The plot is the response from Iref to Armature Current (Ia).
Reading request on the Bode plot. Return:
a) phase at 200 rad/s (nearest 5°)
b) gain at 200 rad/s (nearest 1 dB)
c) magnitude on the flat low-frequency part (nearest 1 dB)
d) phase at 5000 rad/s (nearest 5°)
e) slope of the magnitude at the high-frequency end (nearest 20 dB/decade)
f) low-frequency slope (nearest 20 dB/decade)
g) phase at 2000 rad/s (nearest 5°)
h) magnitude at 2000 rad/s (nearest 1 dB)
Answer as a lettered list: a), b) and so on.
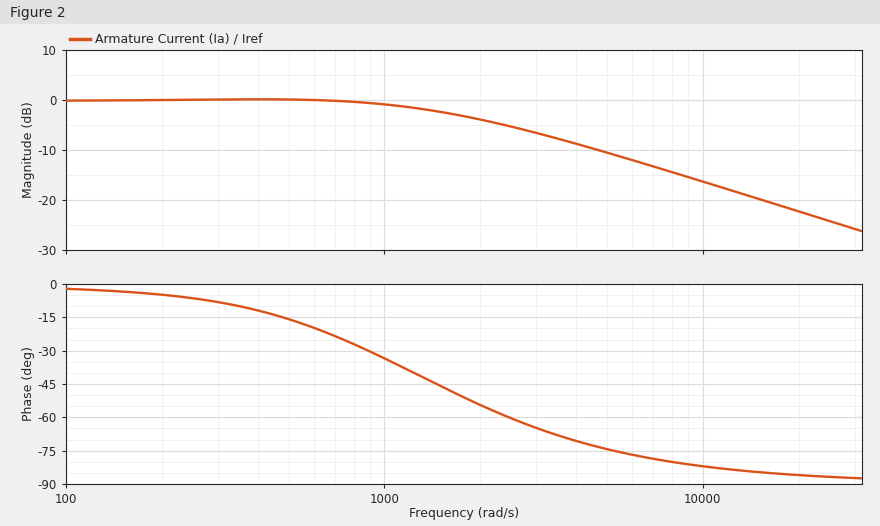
a) -5°
b) 0 dB
c) 0 dB
d) -75°
e) -20 dB/decade
f) 0 dB/decade
g) -55°
h) -4 dB
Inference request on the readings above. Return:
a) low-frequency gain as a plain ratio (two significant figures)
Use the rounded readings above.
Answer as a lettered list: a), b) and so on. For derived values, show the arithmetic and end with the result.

a) 10^(0 / 20) = 1.0
